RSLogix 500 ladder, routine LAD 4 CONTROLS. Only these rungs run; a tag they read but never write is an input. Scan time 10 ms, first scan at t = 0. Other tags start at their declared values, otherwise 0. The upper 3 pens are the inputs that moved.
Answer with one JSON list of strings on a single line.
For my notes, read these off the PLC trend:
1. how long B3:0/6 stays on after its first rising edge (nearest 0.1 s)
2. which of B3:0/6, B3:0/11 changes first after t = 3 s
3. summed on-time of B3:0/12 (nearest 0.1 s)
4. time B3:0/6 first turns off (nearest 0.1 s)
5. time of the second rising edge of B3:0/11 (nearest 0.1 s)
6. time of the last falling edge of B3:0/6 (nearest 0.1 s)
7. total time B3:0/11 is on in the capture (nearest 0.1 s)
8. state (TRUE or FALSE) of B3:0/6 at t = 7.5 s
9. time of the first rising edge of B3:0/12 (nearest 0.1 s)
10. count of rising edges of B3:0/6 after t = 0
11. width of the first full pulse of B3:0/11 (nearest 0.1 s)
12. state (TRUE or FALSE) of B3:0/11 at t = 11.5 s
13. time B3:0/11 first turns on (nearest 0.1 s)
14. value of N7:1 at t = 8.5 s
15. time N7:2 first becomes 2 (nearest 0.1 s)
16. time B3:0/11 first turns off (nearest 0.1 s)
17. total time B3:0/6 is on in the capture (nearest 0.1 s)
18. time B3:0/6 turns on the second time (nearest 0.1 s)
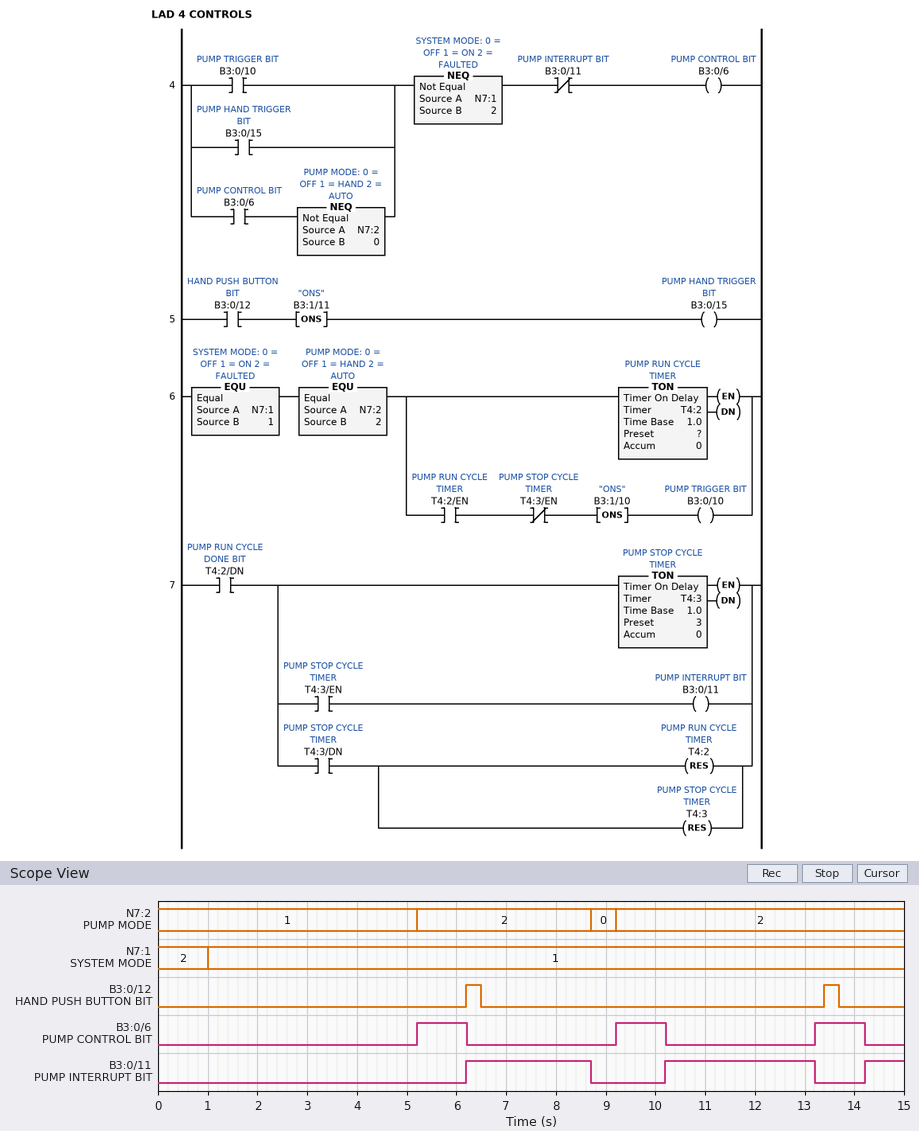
["1.0 s", "B3:0/6", "0.6 s", "6.2 s", "10.2 s", "14.2 s", "6.3 s", "FALSE", "6.2 s", "3", "2.5 s", "TRUE", "6.2 s", "1", "5.2 s", "8.7 s", "3.0 s", "9.2 s"]
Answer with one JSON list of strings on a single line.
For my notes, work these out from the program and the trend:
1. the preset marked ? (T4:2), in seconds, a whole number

["1 s"]
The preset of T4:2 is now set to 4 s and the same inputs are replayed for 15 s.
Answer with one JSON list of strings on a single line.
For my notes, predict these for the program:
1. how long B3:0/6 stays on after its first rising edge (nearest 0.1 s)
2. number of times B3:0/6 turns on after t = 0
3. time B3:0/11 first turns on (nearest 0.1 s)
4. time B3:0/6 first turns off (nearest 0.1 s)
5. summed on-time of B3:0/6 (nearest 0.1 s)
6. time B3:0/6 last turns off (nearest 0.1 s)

["3.5 s", "2", "13.2 s", "8.7 s", "7.5 s", "13.2 s"]
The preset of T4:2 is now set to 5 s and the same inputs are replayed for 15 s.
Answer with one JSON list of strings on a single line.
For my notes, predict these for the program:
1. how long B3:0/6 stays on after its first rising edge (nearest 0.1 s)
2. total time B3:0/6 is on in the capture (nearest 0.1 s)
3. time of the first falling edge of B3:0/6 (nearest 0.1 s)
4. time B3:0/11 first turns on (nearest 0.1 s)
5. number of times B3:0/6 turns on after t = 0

["3.5 s", "8.5 s", "8.7 s", "14.2 s", "2"]
